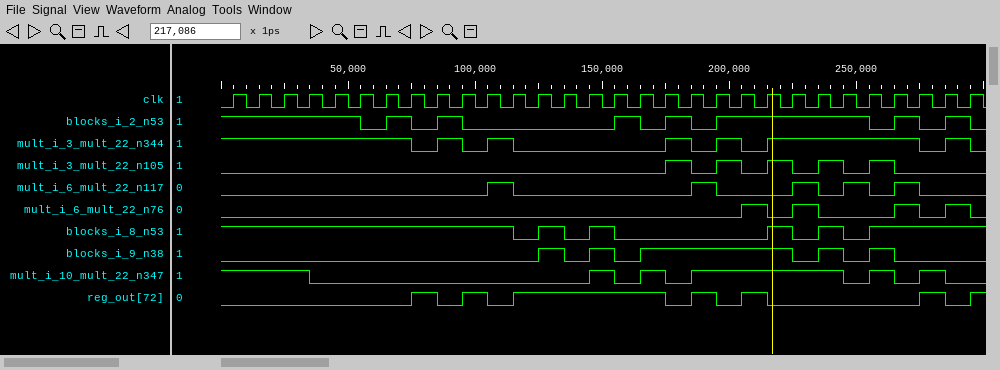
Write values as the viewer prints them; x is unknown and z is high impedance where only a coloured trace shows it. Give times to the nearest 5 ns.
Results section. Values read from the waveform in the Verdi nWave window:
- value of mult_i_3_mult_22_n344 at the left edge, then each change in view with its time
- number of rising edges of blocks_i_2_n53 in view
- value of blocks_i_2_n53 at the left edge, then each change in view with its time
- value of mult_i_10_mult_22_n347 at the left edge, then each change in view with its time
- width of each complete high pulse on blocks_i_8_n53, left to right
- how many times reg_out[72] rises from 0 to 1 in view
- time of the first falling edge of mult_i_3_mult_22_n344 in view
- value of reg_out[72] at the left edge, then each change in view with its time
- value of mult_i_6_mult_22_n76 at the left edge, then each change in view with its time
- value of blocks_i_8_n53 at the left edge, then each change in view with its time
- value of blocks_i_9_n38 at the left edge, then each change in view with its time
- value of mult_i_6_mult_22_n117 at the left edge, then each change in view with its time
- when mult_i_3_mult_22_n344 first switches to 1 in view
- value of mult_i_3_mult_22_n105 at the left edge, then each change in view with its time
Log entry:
1, 0 at 75 ns, 1 at 85 ns, 0 at 95 ns, 1 at 105 ns, 0 at 115 ns, 1 at 175 ns, 0 at 185 ns, 1 at 195 ns, 0 at 205 ns, 1 at 215 ns, 0 at 275 ns, 1 at 285 ns, 0 at 295 ns
7
1, 0 at 55 ns, 1 at 65 ns, 0 at 75 ns, 1 at 85 ns, 0 at 95 ns, 1 at 155 ns, 0 at 165 ns, 1 at 175 ns, 0 at 185 ns, 1 at 195 ns, 0 at 255 ns, 1 at 265 ns, 0 at 275 ns, 1 at 285 ns, 0 at 295 ns
1, 0 at 35 ns, 1 at 145 ns, 0 at 155 ns, 1 at 165 ns, 0 at 175 ns, 1 at 185 ns, 0 at 245 ns, 1 at 255 ns, 0 at 265 ns, 1 at 275 ns, 0 at 285 ns
10 ns, 10 ns, 10 ns, 10 ns
7
75 ns
0, 1 at 75 ns, 0 at 85 ns, 1 at 95 ns, 0 at 105 ns, 1 at 115 ns, 0 at 175 ns, 1 at 185 ns, 0 at 195 ns, 1 at 205 ns, 0 at 215 ns, 1 at 275 ns, 0 at 285 ns, 1 at 295 ns
0, 1 at 205 ns, 0 at 215 ns, 1 at 225 ns, 0 at 235 ns, 1 at 265 ns, 0 at 275 ns, 1 at 285 ns, 0 at 295 ns
1, 0 at 115 ns, 1 at 125 ns, 0 at 135 ns, 1 at 145 ns, 0 at 155 ns, 1 at 215 ns, 0 at 225 ns, 1 at 235 ns, 0 at 245 ns, 1 at 255 ns
0, 1 at 125 ns, 0 at 135 ns, 1 at 145 ns, 0 at 155 ns, 1 at 165 ns, 0 at 225 ns, 1 at 235 ns, 0 at 245 ns, 1 at 255 ns, 0 at 265 ns
0, 1 at 105 ns, 0 at 115 ns, 1 at 185 ns, 0 at 195 ns, 1 at 225 ns, 0 at 235 ns, 1 at 245 ns, 0 at 255 ns, 1 at 265 ns, 0 at 275 ns
85 ns
0, 1 at 175 ns, 0 at 185 ns, 1 at 195 ns, 0 at 205 ns, 1 at 215 ns, 0 at 225 ns, 1 at 235 ns, 0 at 245 ns, 1 at 255 ns, 0 at 265 ns
